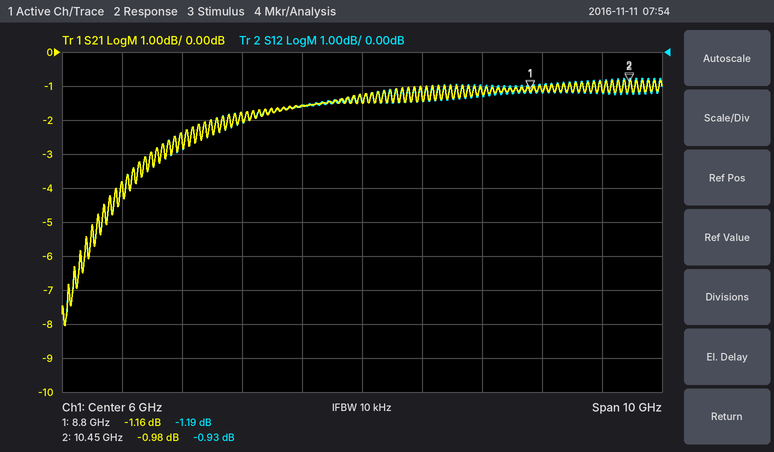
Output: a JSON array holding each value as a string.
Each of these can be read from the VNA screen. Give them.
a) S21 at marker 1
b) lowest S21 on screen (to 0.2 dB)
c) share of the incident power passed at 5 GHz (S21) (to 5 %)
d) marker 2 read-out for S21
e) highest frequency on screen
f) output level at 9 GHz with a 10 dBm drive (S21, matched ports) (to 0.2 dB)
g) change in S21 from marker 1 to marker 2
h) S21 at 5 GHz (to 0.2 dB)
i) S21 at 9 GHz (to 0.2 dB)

["-1.16 dB", "-8.0 dB", "70 %", "-0.98 dB", "11 GHz", "8.8 dBm", "0.18 dB", "-1.6 dB", "-1.2 dB"]
